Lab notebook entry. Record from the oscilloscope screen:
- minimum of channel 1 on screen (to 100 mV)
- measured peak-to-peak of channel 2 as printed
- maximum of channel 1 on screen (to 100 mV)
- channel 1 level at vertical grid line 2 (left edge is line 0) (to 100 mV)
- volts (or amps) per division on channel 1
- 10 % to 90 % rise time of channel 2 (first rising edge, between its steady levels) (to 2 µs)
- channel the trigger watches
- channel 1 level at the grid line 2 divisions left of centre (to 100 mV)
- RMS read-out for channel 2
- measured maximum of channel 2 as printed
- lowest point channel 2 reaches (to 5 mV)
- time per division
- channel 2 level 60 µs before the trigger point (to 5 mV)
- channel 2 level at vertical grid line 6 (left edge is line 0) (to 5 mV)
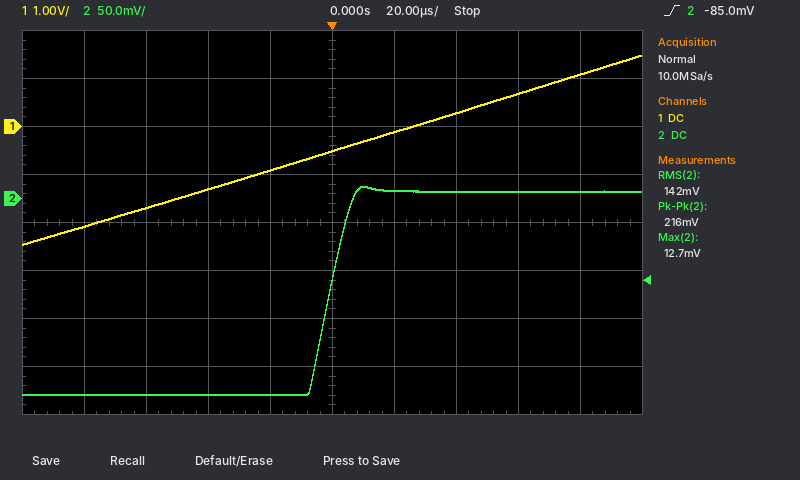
-2.5 V
216 mV
1.5 V
-1.7 V
1 V
12 µs
channel 2
-1.3 V
142 mV
12.7 mV
-205 mV
20 µs
-205 mV
10 mV
